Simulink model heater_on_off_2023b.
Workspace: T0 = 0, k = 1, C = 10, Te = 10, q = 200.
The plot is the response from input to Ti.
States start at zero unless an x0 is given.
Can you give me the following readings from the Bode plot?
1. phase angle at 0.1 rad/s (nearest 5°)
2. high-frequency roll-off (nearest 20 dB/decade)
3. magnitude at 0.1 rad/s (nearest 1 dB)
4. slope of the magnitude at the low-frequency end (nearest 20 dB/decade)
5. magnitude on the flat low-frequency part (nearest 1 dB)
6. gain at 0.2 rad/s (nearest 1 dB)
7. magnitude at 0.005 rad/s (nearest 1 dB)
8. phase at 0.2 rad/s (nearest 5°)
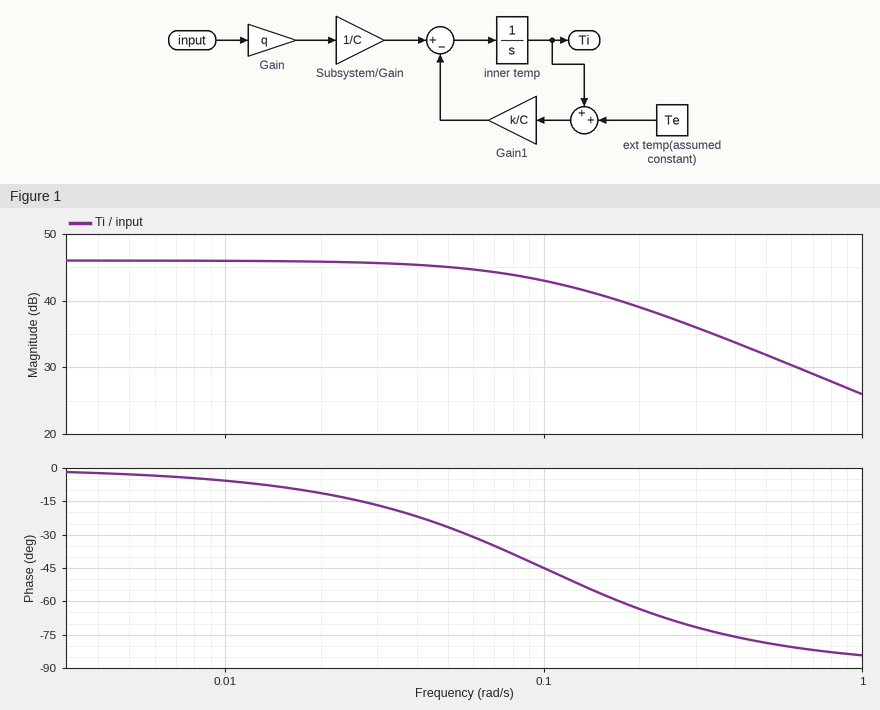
-45°
-20 dB/decade
43 dB
0 dB/decade
46 dB
39 dB
46 dB
-65°
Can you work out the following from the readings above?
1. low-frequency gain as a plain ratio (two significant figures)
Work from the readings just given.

200
